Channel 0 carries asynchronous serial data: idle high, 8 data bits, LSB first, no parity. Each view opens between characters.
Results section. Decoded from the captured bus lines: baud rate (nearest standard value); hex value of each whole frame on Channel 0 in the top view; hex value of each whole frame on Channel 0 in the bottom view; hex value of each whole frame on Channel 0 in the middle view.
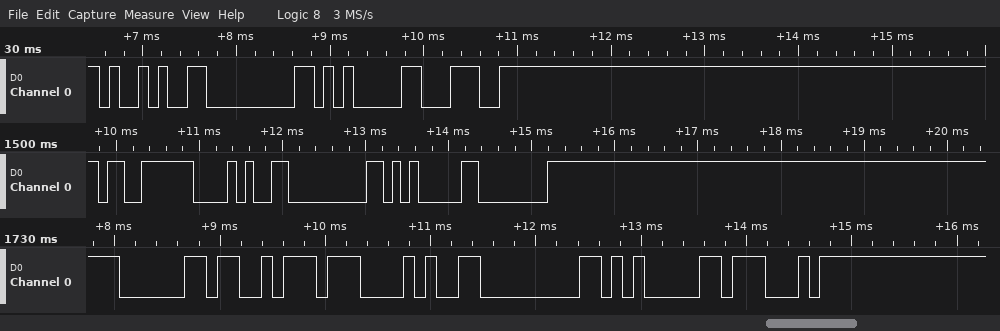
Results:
9600 baud
29, 00, 05, 9C
60, BA, 28, 00, 05, 47
F3, 28, 00, 05, 80
